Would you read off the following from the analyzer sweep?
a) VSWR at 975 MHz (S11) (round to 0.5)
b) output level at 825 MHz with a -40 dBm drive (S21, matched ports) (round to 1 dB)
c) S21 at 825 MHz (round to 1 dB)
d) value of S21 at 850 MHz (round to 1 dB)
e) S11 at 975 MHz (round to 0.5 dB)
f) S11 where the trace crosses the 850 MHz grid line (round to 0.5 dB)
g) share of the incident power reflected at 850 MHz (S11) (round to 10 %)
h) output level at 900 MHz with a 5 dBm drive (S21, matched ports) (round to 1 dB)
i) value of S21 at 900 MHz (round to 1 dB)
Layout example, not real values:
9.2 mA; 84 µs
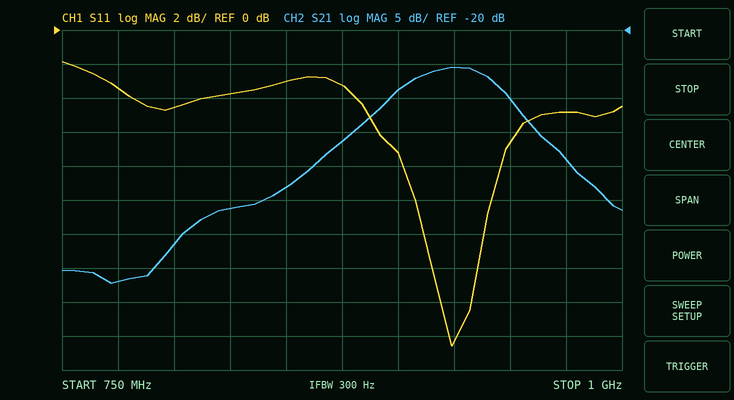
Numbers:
3.5; -86 dBm; -46 dB; -43 dB; -5.0 dB; -3.0 dB; 50 %; -24 dBm; -29 dB
